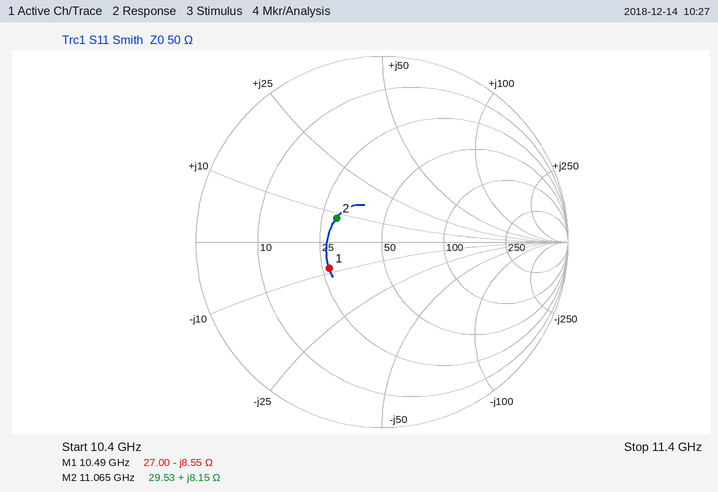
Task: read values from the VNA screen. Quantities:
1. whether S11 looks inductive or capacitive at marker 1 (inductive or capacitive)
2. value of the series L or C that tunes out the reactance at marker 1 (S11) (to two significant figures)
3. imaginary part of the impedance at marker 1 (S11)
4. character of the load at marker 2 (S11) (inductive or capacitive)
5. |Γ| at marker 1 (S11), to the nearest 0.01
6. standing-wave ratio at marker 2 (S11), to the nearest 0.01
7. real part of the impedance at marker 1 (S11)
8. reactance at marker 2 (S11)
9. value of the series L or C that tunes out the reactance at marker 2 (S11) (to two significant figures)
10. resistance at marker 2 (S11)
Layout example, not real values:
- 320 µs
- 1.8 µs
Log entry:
- capacitive
- 130 pH
- -8.55 Ω
- inductive
- 0.32
- 1.76
- 27.00 Ω
- +8.15 Ω
- 1.8 pF
- 29.53 Ω
